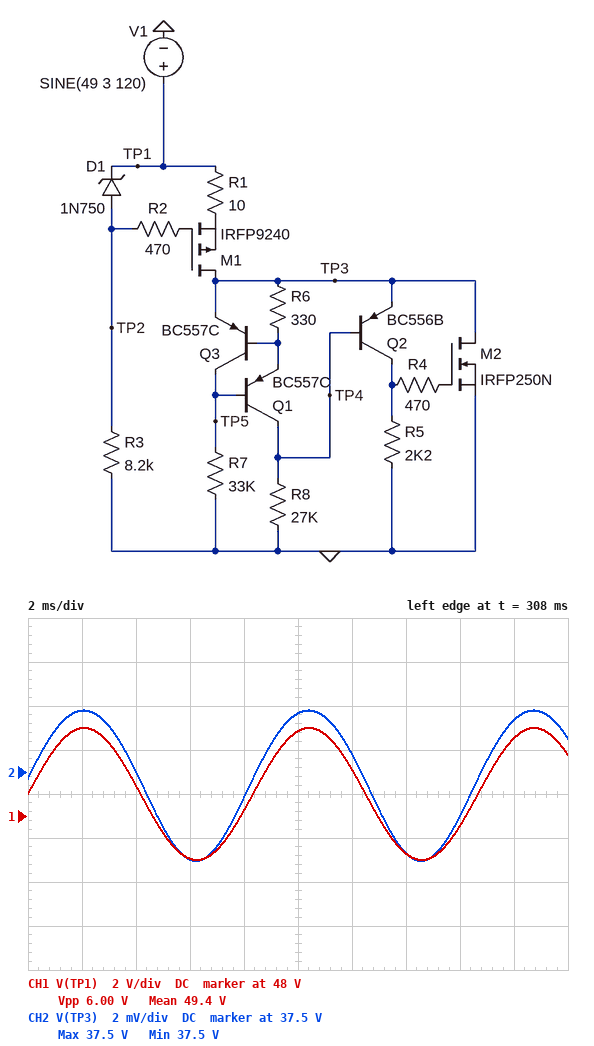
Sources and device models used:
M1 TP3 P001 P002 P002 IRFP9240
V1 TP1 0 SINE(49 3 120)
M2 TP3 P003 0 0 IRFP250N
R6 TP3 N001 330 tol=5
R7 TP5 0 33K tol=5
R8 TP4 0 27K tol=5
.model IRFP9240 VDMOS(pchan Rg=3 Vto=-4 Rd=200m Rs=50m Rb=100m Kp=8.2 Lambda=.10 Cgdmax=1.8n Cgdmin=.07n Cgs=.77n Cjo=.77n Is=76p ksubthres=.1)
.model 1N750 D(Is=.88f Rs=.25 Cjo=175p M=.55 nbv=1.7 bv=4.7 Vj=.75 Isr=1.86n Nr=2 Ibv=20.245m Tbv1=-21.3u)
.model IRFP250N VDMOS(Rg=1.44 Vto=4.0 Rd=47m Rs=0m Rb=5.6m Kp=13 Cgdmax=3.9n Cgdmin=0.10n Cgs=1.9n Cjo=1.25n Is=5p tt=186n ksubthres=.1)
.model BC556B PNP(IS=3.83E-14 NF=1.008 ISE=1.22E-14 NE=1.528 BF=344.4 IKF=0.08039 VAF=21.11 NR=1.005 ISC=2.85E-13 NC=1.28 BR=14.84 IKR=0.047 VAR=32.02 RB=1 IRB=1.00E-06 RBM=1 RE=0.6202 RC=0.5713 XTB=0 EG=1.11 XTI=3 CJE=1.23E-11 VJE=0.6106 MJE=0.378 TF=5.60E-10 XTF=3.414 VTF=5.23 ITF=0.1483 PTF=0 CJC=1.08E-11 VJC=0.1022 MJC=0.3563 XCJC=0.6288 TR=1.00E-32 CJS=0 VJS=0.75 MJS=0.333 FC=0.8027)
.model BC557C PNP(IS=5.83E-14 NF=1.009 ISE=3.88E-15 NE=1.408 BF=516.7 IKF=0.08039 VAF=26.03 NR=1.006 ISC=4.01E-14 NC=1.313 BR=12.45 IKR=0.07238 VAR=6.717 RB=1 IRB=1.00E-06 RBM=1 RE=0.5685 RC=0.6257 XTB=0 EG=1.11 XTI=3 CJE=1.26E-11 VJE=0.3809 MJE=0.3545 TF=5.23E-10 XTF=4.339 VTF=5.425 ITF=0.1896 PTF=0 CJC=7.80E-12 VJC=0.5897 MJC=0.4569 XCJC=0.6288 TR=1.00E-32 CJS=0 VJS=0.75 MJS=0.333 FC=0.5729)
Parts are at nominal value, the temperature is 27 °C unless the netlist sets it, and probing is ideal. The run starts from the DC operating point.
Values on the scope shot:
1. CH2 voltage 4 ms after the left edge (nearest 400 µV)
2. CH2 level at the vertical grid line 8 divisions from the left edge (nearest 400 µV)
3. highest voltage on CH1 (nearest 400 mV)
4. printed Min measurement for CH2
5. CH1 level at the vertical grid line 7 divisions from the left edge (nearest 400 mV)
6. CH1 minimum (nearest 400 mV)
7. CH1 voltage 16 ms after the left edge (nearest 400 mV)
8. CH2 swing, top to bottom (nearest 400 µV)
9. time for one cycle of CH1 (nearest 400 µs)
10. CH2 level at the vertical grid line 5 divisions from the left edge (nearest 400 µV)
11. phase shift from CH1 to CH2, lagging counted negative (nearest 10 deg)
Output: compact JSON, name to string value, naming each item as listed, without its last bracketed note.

{"CH2 voltage 4 ms after the left edge": "37.4980 V", "CH2 level at the vertical grid line 8 divisions from the left edge": "37.4960 V", "highest voltage on CH1": "52.0 V", "printed Min measurement for CH2": "37.5 V", "CH1 level at the vertical grid line 7 divisions from the left edge": "46.4 V", "CH1 minimum": "46.0 V", "CH1 voltage 16 ms after the left edge": "47.6 V", "CH2 swing, top to bottom": "6.8 mV", "time for one cycle of CH1": "8.4 ms", "CH2 level at the vertical grid line 5 divisions from the left edge": "37.5008 V", "phase shift from CH1 to CH2, lagging counted negative": "0 deg"}
